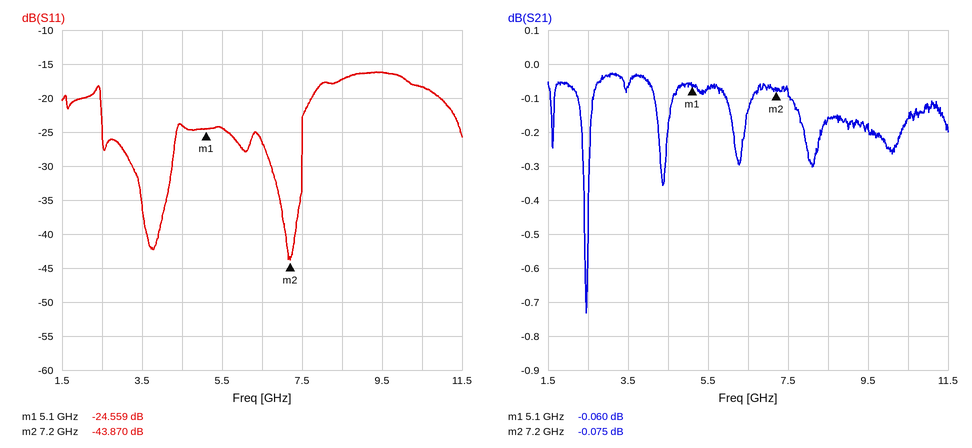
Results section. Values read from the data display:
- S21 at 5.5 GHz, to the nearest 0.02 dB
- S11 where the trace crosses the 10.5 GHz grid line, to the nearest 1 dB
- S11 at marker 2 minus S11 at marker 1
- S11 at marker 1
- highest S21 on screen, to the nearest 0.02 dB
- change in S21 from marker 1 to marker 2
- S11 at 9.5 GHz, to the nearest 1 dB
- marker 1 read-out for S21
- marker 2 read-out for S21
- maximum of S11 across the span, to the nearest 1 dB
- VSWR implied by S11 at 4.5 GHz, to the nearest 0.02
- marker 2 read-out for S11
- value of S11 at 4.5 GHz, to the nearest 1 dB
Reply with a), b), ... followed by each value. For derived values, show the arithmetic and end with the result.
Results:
a) -0.06 dB
b) -18 dB
c) -43.87 − (-24.559) = -19.311 dB
d) -24.559 dB
e) -0.02 dB
f) -0.075 − (-0.06) = -0.015 dB
g) -16 dB
h) -0.060 dB
i) -0.075 dB
j) -16 dB
k) |Γ| = 10^(-24/20) = 0.0631; VSWR = (1 + 0.0631)/(1 − 0.0631) ≈ 1.13, so 1.14 to the nearest 0.02
l) -43.870 dB
m) -24 dB
